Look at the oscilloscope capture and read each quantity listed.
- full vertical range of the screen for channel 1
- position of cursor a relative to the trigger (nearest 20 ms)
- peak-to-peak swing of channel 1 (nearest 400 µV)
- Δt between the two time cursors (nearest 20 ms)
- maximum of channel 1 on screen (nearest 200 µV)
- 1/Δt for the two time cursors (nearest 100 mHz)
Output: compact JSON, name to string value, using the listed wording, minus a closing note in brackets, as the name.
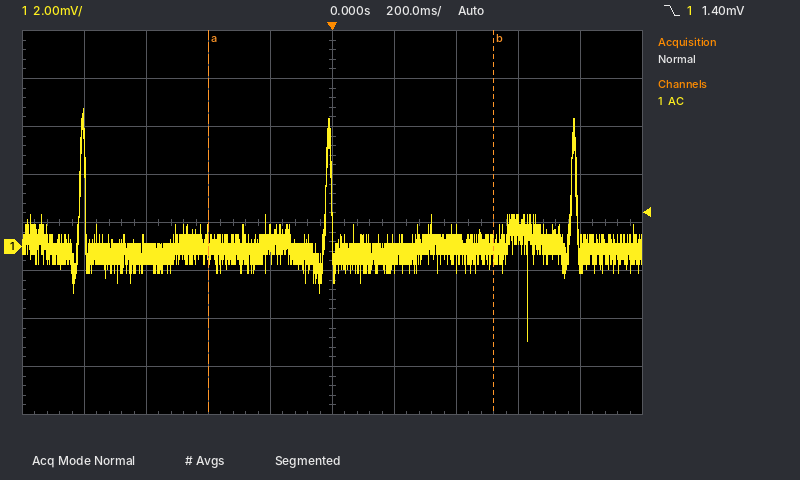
{"full vertical range of the screen for channel 1": "16 mV", "position of cursor a relative to the trigger": "-400 ms", "peak-to-peak swing of channel 1": "9.6 mV", "Δt between the two time cursors": "920 ms", "maximum of channel 1 on screen": "5.8 mV", "1/Δt for the two time cursors": "1.1 Hz"}
